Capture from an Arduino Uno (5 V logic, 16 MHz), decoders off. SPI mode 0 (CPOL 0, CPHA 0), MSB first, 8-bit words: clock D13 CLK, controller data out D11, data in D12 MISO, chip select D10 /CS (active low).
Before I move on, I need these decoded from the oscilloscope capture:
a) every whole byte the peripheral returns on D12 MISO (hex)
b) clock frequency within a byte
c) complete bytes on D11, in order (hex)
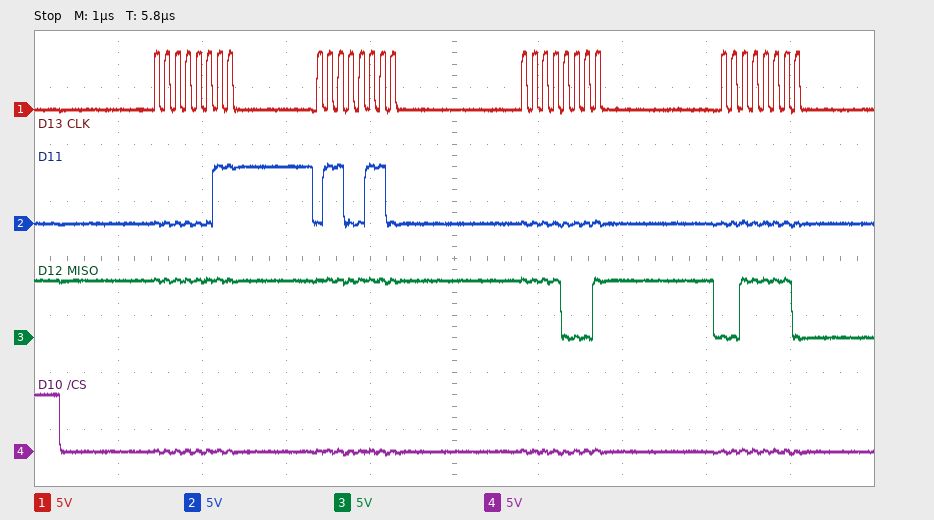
FF FF F1 3E
8 MHz
03 66 00 00
